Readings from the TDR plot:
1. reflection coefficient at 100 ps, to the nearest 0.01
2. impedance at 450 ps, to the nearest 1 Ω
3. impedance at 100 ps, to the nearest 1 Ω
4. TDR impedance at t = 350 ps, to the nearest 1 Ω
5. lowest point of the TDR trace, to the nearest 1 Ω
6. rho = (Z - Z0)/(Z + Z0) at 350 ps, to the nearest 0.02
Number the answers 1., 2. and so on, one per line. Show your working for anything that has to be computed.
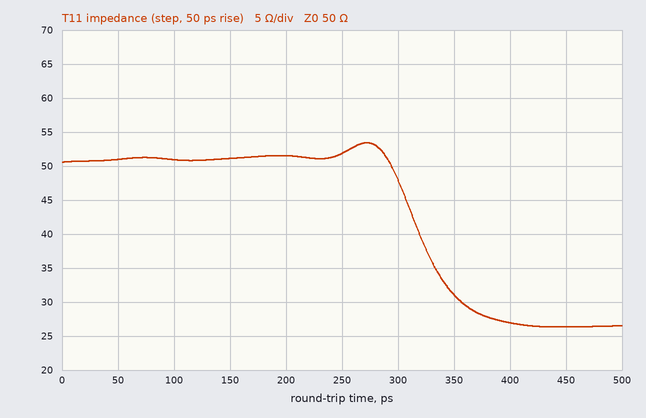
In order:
1. (51 − 50)/(51 + 50) ≈ +0.01
2. 26 Ω
3. 51 Ω
4. 31 Ω
5. 26 Ω
6. (31 − 50)/(31 + 50) ≈ -0.24
